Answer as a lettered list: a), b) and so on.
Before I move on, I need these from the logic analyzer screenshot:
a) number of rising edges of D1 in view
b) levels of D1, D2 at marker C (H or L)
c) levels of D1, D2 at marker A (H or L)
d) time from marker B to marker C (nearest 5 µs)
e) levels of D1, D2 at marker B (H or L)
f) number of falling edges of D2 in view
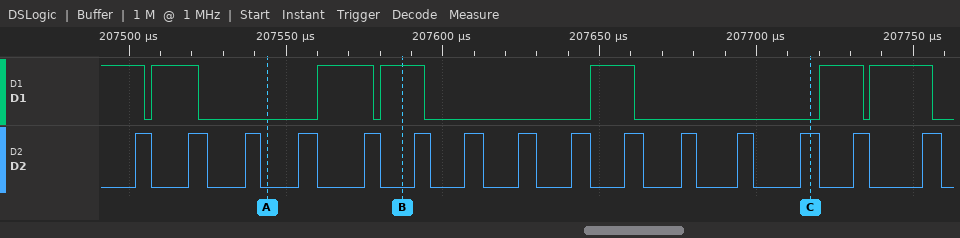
a) 6
b) D1=L, D2=H
c) D1=L, D2=L
d) 130 µs
e) D1=H, D2=L
f) 15
